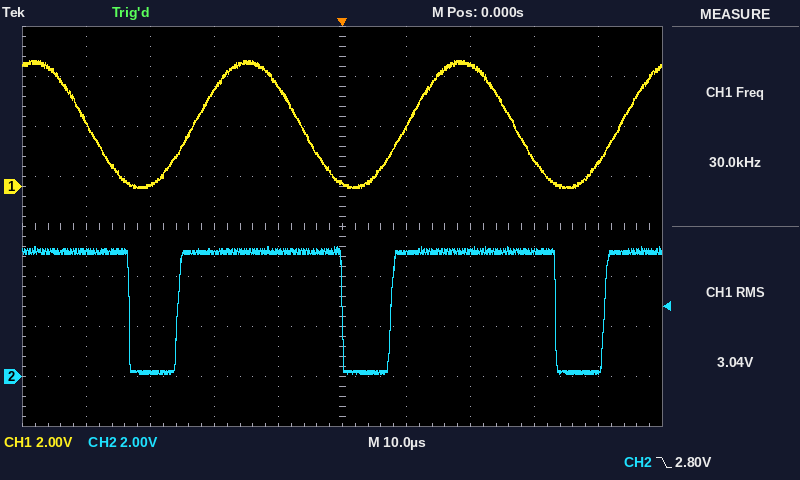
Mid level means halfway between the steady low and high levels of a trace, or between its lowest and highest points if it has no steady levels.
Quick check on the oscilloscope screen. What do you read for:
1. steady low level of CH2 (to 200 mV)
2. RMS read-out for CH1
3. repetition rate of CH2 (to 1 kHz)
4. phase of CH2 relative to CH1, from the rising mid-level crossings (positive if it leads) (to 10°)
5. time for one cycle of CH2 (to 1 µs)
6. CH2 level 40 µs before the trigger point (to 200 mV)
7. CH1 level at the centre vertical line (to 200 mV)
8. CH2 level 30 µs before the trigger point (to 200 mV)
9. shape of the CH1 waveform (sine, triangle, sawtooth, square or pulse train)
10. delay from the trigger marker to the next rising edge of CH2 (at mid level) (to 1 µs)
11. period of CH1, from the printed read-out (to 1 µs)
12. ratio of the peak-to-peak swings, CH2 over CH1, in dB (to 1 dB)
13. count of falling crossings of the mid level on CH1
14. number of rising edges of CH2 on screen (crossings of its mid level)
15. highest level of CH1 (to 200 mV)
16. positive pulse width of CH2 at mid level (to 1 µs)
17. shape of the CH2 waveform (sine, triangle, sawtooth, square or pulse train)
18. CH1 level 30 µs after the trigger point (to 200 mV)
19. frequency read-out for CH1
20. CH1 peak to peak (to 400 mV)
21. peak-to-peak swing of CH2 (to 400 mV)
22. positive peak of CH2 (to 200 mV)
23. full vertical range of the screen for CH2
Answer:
200 mV
3.04 V
30 kHz
+30°
33 µs
5.0 V
200 mV
200 mV
sine
8 µs
33 µs
0 dB
3
3
5.0 V
26 µs
pulse train
1.0 V
30.0 kHz
5.2 V
5.2 V
5.2 V
16 V
